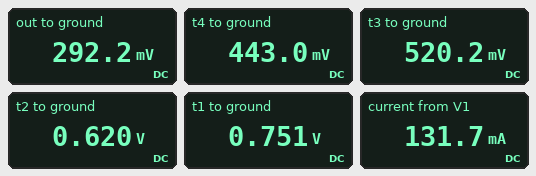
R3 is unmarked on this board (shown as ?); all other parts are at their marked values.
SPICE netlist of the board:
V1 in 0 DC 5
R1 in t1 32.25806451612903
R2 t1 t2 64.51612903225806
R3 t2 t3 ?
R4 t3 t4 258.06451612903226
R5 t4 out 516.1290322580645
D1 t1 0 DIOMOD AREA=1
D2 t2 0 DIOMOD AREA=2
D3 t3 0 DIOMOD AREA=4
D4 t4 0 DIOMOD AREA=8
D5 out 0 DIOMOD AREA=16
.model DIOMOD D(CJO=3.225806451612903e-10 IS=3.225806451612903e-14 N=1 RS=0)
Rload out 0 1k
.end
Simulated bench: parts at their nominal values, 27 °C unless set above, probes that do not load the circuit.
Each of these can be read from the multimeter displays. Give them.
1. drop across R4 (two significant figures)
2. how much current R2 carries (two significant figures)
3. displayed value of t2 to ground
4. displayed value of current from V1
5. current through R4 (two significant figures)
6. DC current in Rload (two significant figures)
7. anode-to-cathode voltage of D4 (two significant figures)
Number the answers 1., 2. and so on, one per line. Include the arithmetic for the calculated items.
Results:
1. 520.2 mV - 443 mV = 77 mV
2. (751 mV - 620 mV) / 64.52 Ω = 2.0 mA
3. 0.620 V
4. 131.7 mA
5. (520.2 mV - 443 mV) / 258.1 Ω = 300 µA
6. (292.2 mV) / 1 kΩ = 290 µA
7. 443 mV = 440 mV
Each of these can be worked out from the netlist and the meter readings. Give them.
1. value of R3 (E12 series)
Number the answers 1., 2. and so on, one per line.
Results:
1. 270 Ω
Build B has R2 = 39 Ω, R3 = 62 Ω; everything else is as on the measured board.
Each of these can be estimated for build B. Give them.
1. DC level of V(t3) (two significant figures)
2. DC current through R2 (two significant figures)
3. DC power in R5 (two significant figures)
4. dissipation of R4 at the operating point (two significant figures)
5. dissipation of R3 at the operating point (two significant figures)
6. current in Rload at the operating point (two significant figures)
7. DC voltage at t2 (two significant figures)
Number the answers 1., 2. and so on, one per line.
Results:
1. 570 mV
2. 3.1 mA
3. 52 µW
4. 32 µW
5. 49 µW
6. 320 µA
7. 630 mV
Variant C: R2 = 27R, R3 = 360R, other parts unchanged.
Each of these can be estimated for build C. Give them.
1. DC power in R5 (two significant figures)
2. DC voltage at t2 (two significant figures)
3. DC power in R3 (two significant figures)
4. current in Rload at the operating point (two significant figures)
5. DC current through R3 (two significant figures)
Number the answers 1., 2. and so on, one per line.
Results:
1. 43 µW
2. 640 mV
3. 44 µW
4. 290 µA
5. 350 µA
